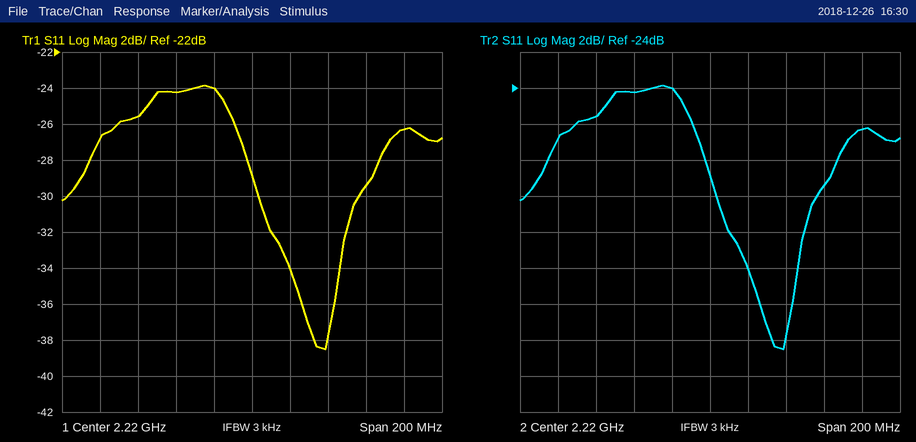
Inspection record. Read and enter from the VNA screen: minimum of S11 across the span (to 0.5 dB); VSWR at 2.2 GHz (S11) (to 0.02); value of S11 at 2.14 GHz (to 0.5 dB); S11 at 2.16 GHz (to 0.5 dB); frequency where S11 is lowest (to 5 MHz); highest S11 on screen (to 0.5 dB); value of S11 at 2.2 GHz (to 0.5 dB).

-38.5 dB
1.14
-27.0 dB
-25.5 dB
2.260 GHz
-24.0 dB
-24.0 dB
